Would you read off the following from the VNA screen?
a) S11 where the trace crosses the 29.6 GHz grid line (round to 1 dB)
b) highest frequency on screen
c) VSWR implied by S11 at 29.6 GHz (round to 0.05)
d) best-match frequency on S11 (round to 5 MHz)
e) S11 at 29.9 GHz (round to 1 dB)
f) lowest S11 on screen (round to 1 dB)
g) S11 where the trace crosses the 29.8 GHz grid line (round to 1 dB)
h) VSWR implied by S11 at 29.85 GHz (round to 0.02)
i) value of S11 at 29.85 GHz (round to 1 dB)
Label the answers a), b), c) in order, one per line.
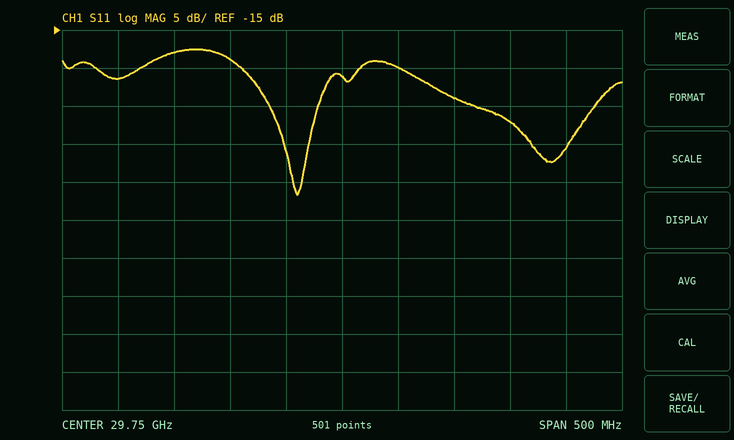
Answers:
a) -18 dB
b) 30 GHz
c) 1.30
d) 29.710 GHz
e) -27 dB
f) -37 dB
g) -20 dB
h) 1.14
i) -24 dB
